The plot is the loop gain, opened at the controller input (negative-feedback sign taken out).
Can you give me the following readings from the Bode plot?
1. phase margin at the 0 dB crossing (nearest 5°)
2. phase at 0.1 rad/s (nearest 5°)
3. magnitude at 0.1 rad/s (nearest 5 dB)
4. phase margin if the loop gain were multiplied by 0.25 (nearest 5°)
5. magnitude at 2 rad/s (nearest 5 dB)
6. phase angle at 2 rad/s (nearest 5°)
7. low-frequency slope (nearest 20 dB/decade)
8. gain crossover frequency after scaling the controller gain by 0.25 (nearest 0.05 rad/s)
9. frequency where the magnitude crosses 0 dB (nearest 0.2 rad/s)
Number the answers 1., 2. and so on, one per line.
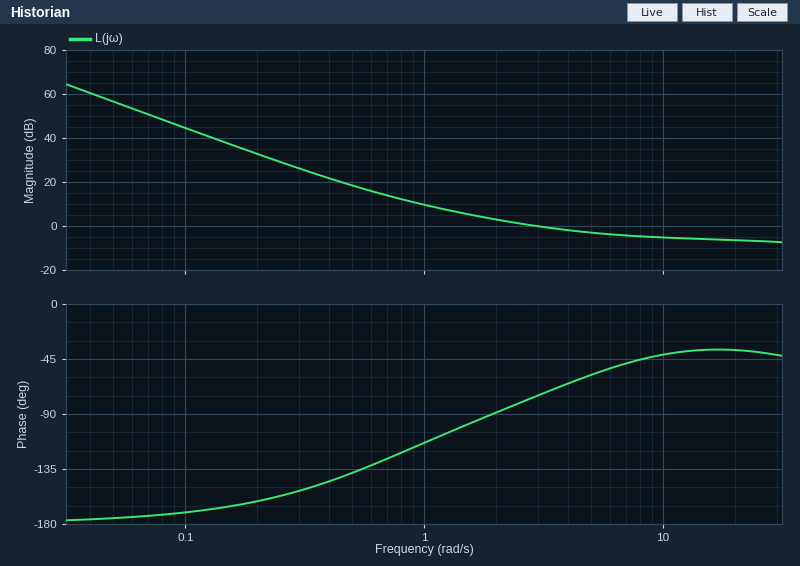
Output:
1. 105°
2. -170°
3. 45 dB
4. 60°
5. 5 dB
6. -90°
7. -40 dB/decade
8. 0.80 rad/s
9. 3.0 rad/s
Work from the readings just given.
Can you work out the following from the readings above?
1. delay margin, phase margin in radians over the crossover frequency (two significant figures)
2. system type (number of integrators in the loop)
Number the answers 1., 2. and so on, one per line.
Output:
1. 0.61 s
2. 2
